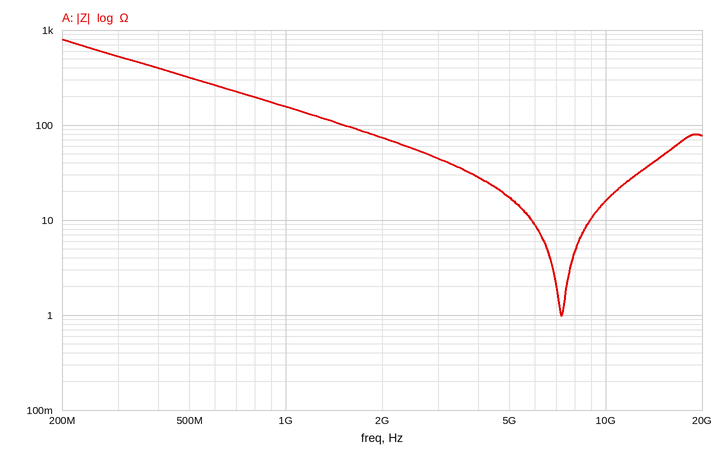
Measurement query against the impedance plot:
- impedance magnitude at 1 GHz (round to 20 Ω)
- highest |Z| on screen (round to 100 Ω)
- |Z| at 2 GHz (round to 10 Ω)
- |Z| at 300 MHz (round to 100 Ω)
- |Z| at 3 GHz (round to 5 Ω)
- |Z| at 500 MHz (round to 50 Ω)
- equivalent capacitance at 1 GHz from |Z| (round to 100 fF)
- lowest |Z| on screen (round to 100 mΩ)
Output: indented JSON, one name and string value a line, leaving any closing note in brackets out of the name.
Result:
{
  "impedance magnitude at 1 GHz": "160 Ω",
  "highest |Z| on screen": "800 Ω",
  "|Z| at 2 GHz": "70 Ω",
  "|Z| at 300 MHz": "500 Ω",
  "|Z| at 3 GHz": "45 Ω",
  "|Z| at 500 MHz": "300 Ω",
  "equivalent capacitance at 1 GHz from |Z|": "1.0 pF",
  "lowest |Z| on screen": "1.0 Ω"
}
